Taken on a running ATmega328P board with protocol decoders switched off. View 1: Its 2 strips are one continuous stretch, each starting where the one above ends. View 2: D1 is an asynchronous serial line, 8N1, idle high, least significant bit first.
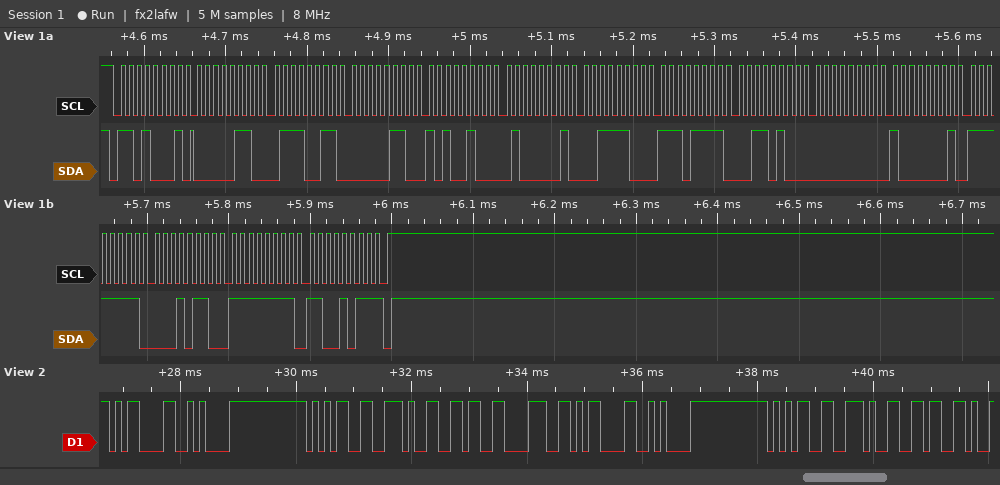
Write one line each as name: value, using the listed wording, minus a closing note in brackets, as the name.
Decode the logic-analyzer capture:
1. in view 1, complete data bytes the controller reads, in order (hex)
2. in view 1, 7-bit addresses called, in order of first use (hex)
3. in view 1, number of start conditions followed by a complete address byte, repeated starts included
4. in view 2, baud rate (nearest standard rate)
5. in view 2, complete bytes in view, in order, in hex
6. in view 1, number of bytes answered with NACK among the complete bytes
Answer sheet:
in view 1, complete data bytes the controller reads, in order: 06 73 06 A4 41 3C EF 34 00 81 FF 16 FF CB
in view 1, 7-bit addresses called, in order of first use: 0x68
in view 1, number of start conditions followed by a complete address byte, repeated starts included: 1
in view 2, baud rate: 9600 baud
in view 2, complete bytes in view, in order, in hex: 0D 0A 35 2E 36 38 0D 0A 35 2E 36
in view 1, number of bytes answered with NACK among the complete bytes: 1
